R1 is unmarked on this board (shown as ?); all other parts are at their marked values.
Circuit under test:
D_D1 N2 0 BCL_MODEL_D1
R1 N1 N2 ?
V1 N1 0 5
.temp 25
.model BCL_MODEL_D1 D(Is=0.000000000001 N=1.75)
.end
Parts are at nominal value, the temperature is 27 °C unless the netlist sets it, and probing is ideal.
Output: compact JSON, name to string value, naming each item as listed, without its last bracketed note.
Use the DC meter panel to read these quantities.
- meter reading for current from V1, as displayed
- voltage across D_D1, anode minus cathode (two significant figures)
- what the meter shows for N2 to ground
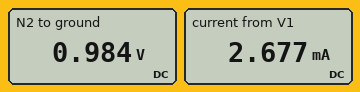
{"meter reading for current from V1, as displayed": "2.677 mA", "voltage across D_D1, anode minus cathode": "980 mV", "what the meter shows for N2 to ground": "0.984 V"}
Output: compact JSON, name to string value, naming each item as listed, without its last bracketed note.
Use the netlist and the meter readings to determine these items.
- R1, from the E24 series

{"R1, from the E24 series": "1.5 kΩ"}
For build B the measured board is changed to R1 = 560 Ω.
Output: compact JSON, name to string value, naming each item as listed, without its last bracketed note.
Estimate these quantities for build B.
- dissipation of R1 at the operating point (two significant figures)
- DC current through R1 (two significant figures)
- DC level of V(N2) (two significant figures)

{"dissipation of R1 at the operating point": "28 mW", "DC current through R1": "7.1 mA", "DC level of V(N2)": "1.0 V"}
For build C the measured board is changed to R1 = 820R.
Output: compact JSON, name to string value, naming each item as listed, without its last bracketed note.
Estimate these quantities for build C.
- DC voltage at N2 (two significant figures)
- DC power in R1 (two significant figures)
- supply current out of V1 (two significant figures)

{"DC voltage at N2": "1.0 V", "DC power in R1": "19 mW", "supply current out of V1": "4.9 mA"}
